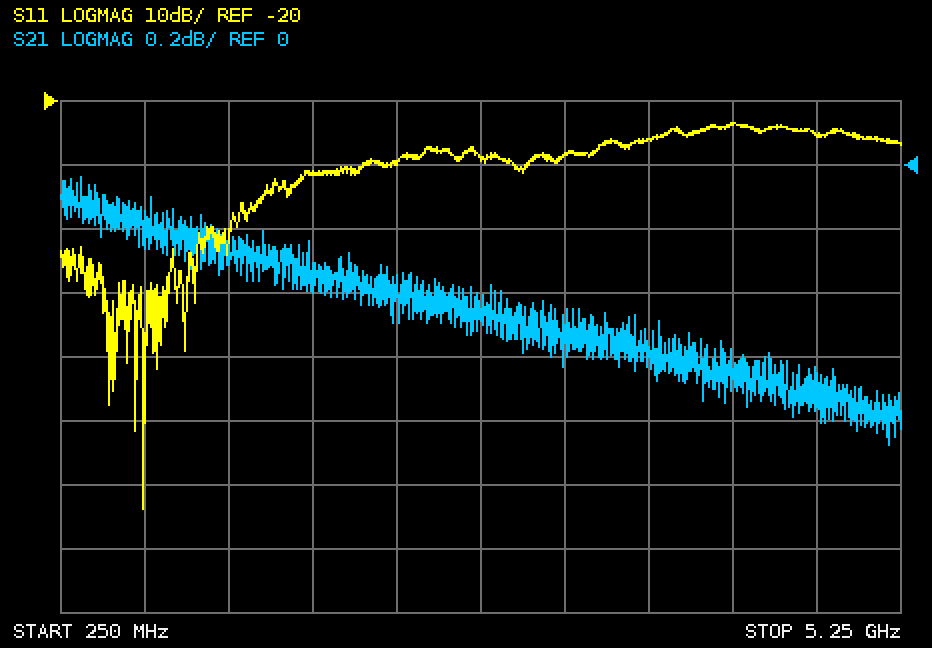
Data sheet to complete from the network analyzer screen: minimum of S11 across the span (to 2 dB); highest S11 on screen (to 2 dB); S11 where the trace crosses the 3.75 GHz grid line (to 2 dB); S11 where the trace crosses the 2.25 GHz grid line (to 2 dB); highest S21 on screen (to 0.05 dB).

-84 dB
-24 dB
-26 dB
-30 dB
-0.05 dB
